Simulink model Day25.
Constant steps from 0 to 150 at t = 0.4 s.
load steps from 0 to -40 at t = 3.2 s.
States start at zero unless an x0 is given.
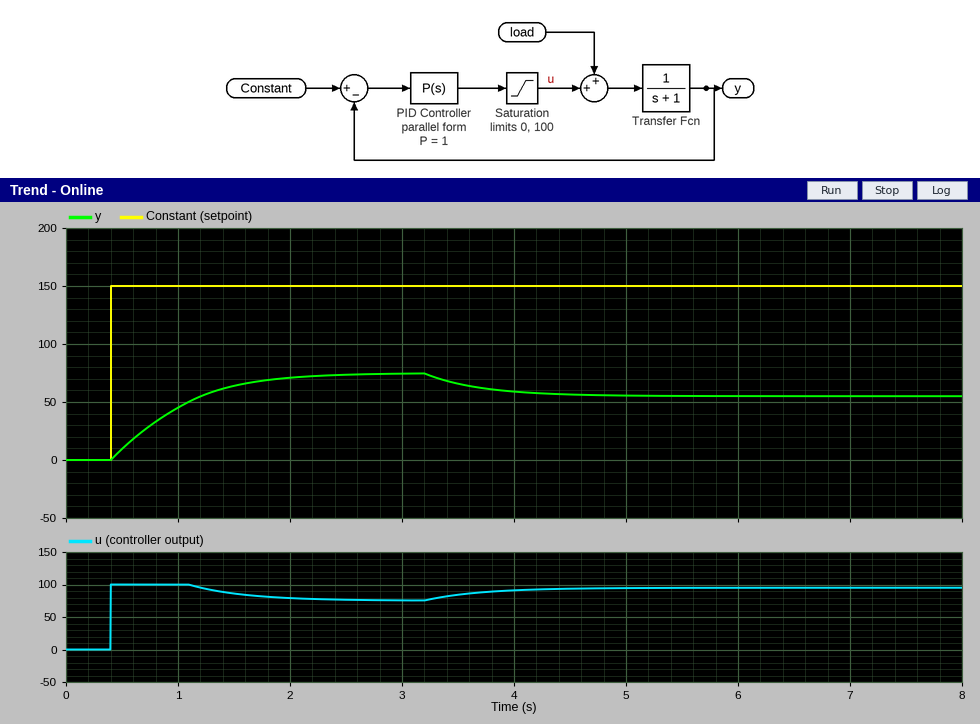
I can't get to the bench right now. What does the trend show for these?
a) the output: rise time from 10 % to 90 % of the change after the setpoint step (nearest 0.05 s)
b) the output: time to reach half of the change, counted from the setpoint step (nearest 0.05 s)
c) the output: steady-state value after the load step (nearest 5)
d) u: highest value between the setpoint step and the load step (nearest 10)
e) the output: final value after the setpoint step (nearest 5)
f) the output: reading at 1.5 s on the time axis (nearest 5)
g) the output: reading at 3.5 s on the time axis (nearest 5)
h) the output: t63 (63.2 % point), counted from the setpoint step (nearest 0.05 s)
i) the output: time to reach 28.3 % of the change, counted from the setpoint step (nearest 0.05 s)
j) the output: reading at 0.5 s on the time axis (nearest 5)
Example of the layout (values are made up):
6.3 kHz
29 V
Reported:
1.20 s
0.45 s
55
100
75
65
65
0.65 s
0.25 s
10
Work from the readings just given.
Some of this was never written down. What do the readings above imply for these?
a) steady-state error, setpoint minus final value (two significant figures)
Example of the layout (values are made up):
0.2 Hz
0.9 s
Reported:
75
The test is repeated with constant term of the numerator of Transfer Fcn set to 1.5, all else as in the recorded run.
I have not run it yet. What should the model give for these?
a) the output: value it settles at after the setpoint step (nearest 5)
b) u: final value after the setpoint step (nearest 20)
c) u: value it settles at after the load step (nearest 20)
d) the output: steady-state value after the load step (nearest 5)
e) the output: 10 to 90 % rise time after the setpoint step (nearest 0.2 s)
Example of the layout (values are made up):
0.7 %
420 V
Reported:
90
60
80
65
1.0 s
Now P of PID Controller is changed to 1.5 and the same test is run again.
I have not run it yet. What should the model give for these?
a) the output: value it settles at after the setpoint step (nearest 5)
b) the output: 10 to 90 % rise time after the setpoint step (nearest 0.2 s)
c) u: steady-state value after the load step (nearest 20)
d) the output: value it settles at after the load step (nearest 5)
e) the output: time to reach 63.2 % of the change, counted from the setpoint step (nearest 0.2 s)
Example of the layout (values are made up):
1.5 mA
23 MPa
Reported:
90
1.6 s
100
60
0.8 s
